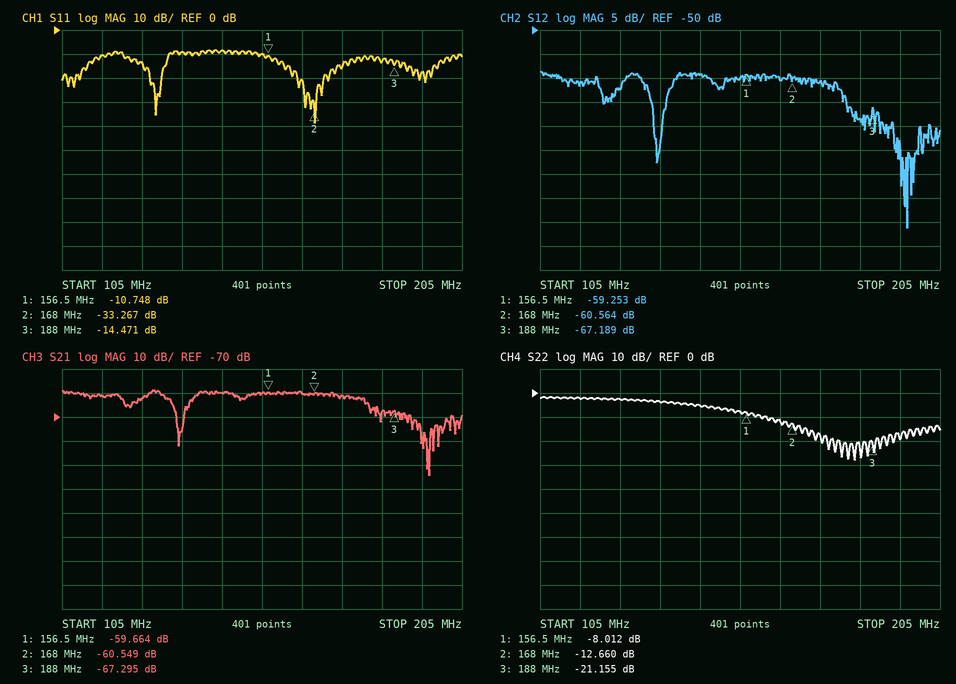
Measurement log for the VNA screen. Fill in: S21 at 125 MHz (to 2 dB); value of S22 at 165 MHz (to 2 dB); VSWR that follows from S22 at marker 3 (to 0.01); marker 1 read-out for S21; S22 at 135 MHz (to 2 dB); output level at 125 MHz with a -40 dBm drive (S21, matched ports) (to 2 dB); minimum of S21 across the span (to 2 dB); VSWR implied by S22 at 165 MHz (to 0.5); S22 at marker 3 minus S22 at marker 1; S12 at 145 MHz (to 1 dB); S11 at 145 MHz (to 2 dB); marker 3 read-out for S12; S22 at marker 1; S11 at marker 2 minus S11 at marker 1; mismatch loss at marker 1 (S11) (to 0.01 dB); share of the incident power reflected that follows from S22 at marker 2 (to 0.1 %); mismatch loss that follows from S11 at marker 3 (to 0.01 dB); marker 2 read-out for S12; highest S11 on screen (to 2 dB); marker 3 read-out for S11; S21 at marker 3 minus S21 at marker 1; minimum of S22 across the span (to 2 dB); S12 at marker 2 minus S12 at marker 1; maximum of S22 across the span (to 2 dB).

-62 dB
-12 dB
1.19
-59.664 dB
-4 dB
-102 dBm
-94 dB
1.5
-13.143 dB
-59 dB
-8 dB
-67.189 dB
-8.012 dB
-22.519 dB
0.38 dB
5.4 %
0.16 dB
-60.564 dB
-8 dB
-14.471 dB
-7.631 dB
-28 dB
-1.311 dB
-2 dB
